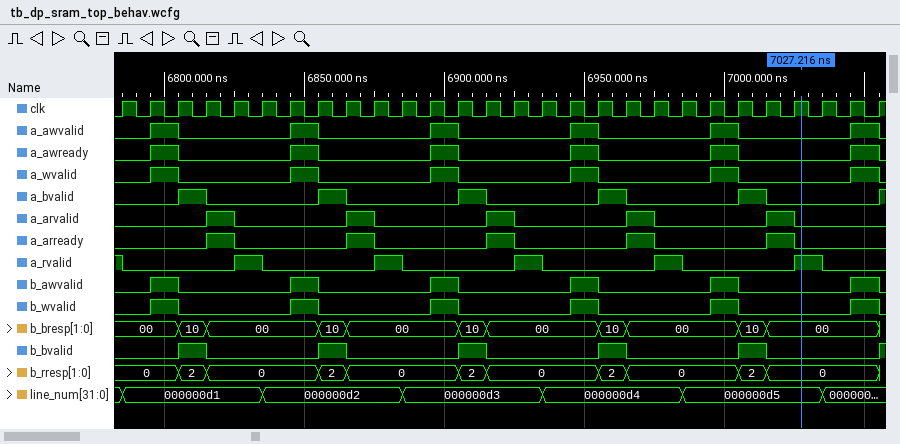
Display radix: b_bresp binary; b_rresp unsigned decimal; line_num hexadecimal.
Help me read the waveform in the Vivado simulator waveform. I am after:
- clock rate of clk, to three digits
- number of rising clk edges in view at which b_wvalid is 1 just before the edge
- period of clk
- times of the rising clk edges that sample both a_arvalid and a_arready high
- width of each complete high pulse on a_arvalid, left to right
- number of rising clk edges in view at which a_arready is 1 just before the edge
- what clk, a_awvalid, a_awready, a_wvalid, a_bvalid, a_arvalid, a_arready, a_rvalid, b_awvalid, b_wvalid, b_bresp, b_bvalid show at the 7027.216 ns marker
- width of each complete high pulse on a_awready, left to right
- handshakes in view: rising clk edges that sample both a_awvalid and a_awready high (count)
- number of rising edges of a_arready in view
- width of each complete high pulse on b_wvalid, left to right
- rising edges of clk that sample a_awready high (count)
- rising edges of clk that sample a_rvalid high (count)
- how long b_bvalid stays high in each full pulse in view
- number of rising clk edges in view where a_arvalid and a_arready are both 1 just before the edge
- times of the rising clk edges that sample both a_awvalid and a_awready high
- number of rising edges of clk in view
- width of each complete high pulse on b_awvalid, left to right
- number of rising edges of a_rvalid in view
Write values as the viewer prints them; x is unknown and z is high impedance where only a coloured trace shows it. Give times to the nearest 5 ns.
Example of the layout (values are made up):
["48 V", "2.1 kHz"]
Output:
["100 MHz", "6", "10 ns", "6825 ns, 6875 ns, 6925 ns, 6975 ns, 7025 ns", "10 ns, 10 ns, 10 ns, 10 ns, 10 ns", "5", "clk=1, a_awvalid=0, a_awready=0, a_wvalid=0, a_bvalid=0, a_arvalid=0, a_arready=0, a_rvalid=1, b_awvalid=0, b_wvalid=0, b_bresp=00, b_bvalid=0", "10 ns, 10 ns, 10 ns, 10 ns, 10 ns, 10 ns", "6", "5", "10 ns, 10 ns, 10 ns, 10 ns, 10 ns, 10 ns", "6", "6", "10 ns, 10 ns, 10 ns, 10 ns, 10 ns", "5", "6805 ns, 6855 ns, 6905 ns, 6955 ns, 7005 ns, 7055 ns", "28", "10 ns, 10 ns, 10 ns, 10 ns, 10 ns, 10 ns", "5"]
